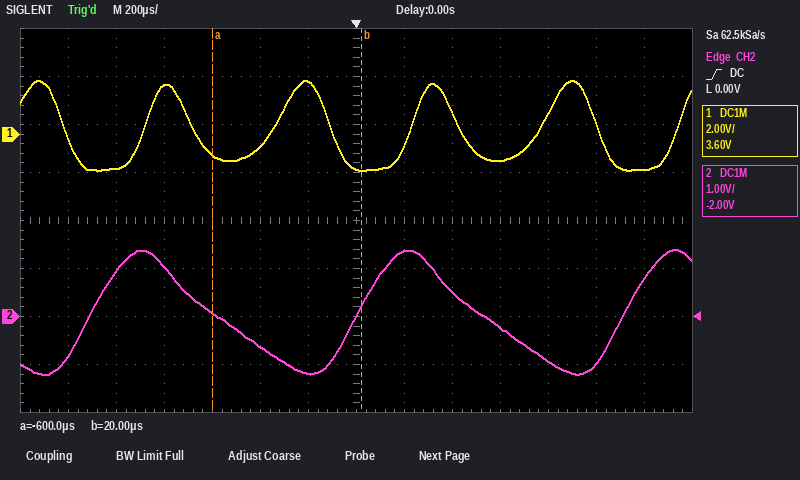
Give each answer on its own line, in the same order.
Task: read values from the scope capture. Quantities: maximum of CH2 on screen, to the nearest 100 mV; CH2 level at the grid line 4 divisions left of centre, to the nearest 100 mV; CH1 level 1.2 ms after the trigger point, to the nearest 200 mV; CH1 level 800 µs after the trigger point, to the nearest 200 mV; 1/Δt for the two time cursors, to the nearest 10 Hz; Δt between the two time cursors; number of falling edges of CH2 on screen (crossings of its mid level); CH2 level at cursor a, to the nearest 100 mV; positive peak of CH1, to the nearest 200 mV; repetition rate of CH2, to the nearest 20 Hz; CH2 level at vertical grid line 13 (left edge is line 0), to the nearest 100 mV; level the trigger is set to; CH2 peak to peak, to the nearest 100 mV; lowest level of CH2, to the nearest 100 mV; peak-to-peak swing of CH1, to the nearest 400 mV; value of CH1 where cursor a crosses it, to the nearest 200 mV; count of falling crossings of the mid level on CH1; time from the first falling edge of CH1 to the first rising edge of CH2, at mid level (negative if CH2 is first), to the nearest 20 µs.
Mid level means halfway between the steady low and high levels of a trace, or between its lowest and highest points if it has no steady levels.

1.4 V
1.0 V
-1.4 V
800 mV
1.61 kHz
620 µs
2
100 mV
2.2 V
900 Hz
800 mV
0.00 V
2.6 V
-1.2 V
3.6 V
-800 mV
5
+120 µs
